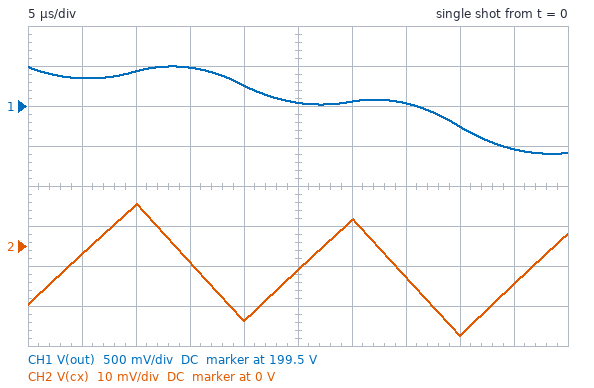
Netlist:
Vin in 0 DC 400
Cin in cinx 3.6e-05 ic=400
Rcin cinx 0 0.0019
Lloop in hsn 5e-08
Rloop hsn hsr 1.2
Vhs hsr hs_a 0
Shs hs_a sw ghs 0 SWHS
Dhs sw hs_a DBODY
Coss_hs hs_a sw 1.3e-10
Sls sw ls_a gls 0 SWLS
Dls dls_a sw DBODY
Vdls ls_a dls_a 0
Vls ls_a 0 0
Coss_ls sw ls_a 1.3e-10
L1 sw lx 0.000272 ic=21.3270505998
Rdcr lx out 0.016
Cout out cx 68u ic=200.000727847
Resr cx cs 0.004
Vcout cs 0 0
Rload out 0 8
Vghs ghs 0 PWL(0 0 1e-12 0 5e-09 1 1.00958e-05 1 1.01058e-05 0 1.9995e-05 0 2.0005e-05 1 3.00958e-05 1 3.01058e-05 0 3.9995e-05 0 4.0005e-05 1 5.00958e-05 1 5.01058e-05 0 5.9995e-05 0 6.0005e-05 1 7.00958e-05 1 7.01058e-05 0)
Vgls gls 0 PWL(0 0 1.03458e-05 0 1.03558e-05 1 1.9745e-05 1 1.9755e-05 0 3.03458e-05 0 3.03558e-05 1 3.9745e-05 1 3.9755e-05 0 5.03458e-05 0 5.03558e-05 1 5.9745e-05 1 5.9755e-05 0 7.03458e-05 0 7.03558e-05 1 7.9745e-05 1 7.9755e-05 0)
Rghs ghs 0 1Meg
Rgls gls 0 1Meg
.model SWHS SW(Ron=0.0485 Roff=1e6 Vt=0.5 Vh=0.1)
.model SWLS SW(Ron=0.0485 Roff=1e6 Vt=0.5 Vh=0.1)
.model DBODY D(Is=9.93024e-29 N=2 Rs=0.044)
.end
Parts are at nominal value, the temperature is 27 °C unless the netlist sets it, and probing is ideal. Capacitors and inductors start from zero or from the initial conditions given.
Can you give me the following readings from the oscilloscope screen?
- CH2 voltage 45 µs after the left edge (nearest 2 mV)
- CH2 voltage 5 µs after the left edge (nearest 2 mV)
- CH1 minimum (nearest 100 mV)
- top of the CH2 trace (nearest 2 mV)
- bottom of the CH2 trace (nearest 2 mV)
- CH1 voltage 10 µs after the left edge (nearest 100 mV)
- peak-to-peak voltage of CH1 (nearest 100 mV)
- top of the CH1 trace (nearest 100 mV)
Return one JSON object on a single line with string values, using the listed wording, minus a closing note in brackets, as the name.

{"CH2 voltage 45 µs after the left edge": "-10 mV", "CH2 voltage 5 µs after the left edge": "-2 mV", "CH1 minimum": "198.9 V", "top of the CH2 trace": "10 mV", "bottom of the CH2 trace": "-22 mV", "CH1 voltage 10 µs after the left edge": "199.9 V", "peak-to-peak voltage of CH1": "1.1 V", "top of the CH1 trace": "200.0 V"}
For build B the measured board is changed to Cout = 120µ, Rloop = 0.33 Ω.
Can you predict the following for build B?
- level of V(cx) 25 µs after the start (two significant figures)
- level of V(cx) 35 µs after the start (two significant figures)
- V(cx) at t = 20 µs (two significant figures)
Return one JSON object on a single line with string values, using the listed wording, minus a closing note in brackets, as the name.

{"level of V(cx) 25 µs after the start": "-1.7 mV", "level of V(cx) 35 µs after the start": "-2.1 mV", "V(cx) at t = 20 µs": "-16 mV"}
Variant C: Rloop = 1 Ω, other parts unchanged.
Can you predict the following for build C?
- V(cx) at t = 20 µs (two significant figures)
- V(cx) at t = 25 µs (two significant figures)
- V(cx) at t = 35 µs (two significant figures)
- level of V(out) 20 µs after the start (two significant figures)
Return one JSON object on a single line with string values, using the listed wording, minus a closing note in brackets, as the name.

{"V(cx) at t = 20 µs": "-18 mV", "V(cx) at t = 25 µs": "-5.0 mV", "V(cx) at t = 35 µs": "-6.5 mV", "level of V(out) 20 µs after the start": "200 V"}
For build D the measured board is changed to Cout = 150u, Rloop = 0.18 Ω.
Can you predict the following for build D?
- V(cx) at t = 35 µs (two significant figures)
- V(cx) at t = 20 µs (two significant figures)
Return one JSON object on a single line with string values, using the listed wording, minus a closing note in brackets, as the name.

{"V(cx) at t = 35 µs": "-1.0 mV", "V(cx) at t = 20 µs": "-15 mV"}
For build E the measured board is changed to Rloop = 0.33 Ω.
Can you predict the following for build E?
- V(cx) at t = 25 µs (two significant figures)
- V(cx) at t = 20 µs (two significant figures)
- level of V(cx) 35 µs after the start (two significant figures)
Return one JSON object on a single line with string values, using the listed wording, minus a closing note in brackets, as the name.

{"V(cx) at t = 25 µs": "-1.7 mV", "V(cx) at t = 20 µs": "-16 mV", "level of V(cx) 35 µs after the start": "-2.0 mV"}
